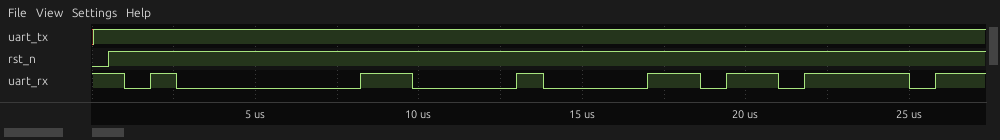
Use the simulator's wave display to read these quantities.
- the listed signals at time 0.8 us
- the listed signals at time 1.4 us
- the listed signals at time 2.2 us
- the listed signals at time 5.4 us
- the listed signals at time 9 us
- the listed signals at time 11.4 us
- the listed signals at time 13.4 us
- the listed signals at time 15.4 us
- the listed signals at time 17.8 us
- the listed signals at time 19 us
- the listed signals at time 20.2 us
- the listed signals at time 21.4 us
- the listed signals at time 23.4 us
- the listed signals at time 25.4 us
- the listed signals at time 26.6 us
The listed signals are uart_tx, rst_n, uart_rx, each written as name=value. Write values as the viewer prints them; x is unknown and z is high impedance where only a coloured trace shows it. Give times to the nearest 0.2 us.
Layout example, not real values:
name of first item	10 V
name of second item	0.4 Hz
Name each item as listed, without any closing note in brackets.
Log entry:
the listed signals at time 0.8 us	uart_tx=1, rst_n=1, uart_rx=1
the listed signals at time 1.4 us	uart_tx=1, rst_n=1, uart_rx=0
the listed signals at time 2.2 us	uart_tx=1, rst_n=1, uart_rx=1
the listed signals at time 5.4 us	uart_tx=1, rst_n=1, uart_rx=0
the listed signals at time 9 us	uart_tx=1, rst_n=1, uart_rx=1
the listed signals at time 11.4 us	uart_tx=1, rst_n=1, uart_rx=0
the listed signals at time 13.4 us	uart_tx=1, rst_n=1, uart_rx=1
the listed signals at time 15.4 us	uart_tx=1, rst_n=1, uart_rx=0
the listed signals at time 17.8 us	uart_tx=1, rst_n=1, uart_rx=1
the listed signals at time 19 us	uart_tx=1, rst_n=1, uart_rx=0
the listed signals at time 20.2 us	uart_tx=1, rst_n=1, uart_rx=1
the listed signals at time 21.4 us	uart_tx=1, rst_n=1, uart_rx=0
the listed signals at time 23.4 us	uart_tx=1, rst_n=1, uart_rx=1
the listed signals at time 25.4 us	uart_tx=1, rst_n=1, uart_rx=0
the listed signals at time 26.6 us	uart_tx=1, rst_n=1, uart_rx=1
